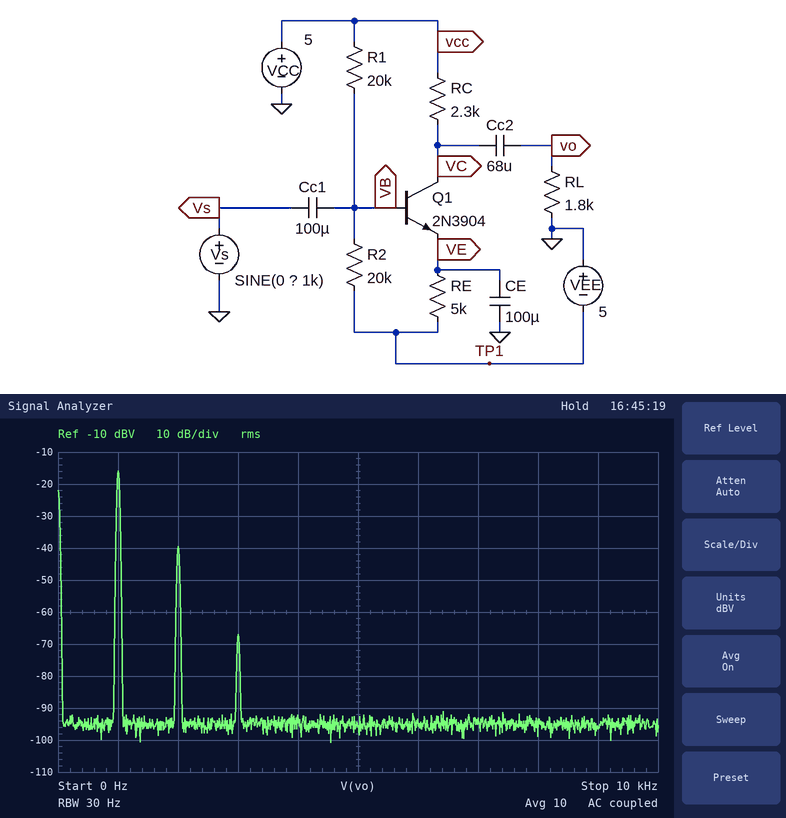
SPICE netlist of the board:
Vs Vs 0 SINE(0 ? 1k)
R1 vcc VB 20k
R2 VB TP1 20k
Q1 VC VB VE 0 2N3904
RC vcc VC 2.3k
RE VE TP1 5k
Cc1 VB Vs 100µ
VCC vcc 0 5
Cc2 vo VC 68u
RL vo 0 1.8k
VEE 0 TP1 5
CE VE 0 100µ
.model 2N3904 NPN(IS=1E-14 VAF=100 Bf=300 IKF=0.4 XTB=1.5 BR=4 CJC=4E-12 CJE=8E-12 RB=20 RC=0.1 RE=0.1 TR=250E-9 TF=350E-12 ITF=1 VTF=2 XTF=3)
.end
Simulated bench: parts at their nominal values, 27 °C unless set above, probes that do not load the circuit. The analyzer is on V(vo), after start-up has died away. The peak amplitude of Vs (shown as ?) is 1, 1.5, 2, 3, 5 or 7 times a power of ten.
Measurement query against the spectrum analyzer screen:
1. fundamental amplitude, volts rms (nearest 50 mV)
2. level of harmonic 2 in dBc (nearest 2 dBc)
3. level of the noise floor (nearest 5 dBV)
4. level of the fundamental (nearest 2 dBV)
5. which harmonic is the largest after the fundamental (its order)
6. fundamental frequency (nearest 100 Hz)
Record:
150 mV
-24 dBc
-95 dBV
-16 dBV
2
1.0 kHz
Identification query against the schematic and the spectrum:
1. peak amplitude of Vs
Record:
7 mV
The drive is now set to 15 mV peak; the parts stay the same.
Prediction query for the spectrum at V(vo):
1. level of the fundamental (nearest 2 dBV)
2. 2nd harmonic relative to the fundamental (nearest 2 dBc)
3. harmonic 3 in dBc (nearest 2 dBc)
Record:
-10 dBV
-18 dBc
-38 dBc
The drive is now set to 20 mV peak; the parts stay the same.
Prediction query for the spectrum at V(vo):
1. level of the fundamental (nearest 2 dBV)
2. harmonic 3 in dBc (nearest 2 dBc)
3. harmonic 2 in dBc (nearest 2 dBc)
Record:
-8 dBV
-34 dBc
-14 dBc
